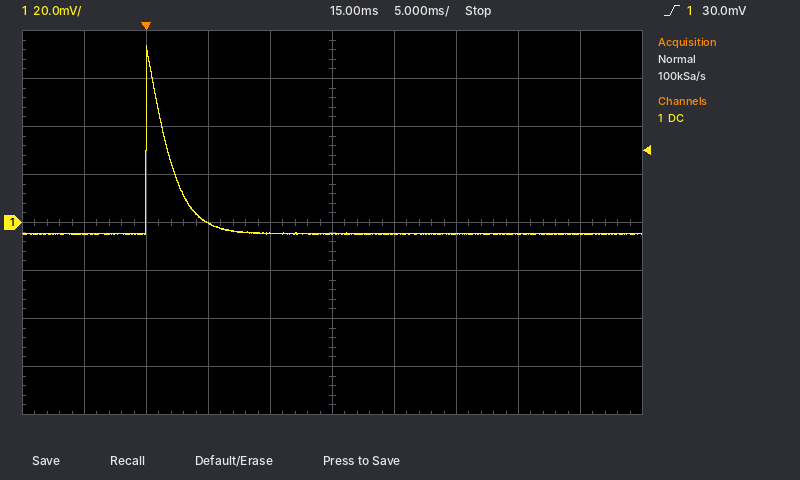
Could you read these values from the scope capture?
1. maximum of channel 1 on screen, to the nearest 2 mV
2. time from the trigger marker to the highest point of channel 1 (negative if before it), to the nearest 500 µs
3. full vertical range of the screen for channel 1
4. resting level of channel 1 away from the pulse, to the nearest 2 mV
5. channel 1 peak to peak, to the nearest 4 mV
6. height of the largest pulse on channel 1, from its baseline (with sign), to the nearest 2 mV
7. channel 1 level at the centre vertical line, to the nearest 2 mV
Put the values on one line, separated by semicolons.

74 mV; 0.0 ms; 160 mV; -4 mV; 80 mV; +78 mV; -4 mV
